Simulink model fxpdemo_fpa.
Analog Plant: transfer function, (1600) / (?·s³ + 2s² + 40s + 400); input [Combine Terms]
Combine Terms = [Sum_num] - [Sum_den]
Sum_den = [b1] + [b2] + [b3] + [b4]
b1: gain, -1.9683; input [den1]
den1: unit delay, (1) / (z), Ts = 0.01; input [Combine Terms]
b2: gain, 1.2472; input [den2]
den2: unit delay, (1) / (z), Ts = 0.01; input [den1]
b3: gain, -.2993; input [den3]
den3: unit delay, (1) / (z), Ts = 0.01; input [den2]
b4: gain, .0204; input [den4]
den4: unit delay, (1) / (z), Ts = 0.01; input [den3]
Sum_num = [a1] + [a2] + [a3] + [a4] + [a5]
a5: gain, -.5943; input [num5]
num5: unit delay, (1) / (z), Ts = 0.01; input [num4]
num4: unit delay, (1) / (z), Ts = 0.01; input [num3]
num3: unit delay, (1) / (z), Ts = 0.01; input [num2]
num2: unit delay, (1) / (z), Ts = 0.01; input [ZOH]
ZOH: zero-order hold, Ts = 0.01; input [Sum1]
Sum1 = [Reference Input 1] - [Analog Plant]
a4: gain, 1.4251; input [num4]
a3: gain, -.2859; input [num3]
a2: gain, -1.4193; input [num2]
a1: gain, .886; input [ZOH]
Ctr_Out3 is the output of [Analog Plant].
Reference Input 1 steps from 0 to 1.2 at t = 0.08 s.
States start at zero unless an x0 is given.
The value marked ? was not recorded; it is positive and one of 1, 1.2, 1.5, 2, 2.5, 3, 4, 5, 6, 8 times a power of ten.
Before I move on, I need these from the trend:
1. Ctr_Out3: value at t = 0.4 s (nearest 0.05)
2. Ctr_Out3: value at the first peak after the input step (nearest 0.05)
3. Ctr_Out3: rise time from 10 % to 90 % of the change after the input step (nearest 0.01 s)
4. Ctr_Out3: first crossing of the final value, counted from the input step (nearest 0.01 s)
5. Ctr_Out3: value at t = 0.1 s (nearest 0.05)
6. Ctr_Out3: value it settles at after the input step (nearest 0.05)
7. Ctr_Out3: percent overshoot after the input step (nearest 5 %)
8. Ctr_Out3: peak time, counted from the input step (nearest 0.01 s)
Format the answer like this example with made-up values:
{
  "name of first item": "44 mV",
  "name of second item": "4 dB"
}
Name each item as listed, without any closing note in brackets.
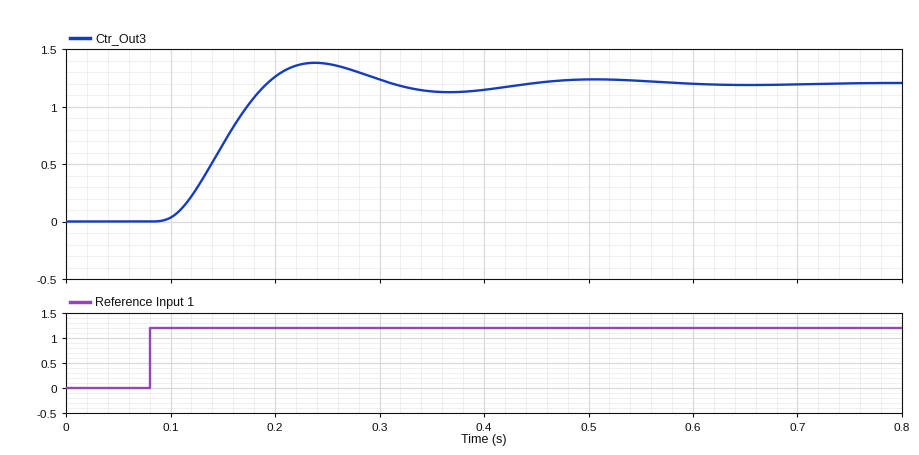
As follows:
{
  "Ctr_Out3: value at t = 0.4 s": "1.15",
  "Ctr_Out3: value at the first peak after the input step": "1.40",
  "Ctr_Out3: rise time from 10 % to 90 % of the change after the input step": "0.07 s",
  "Ctr_Out3: first crossing of the final value, counted from the input step": "0.11 s",
  "Ctr_Out3: value at t = 0.1 s": "0.05",
  "Ctr_Out3: value it settles at after the input step": "1.20",
  "Ctr_Out3: percent overshoot after the input step": "15 %",
  "Ctr_Out3: peak time, counted from the input step": "0.16 s"
}
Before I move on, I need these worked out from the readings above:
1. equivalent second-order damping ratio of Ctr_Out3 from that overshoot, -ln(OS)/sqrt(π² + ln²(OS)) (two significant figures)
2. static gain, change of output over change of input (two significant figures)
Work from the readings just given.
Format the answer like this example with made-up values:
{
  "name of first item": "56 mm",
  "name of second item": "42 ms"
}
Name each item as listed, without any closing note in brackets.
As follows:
{
  "equivalent second-order damping ratio of Ctr_Out3 from that overshoot, -ln(OS)/sqrt(π² + ln²(OS))": "0.52",
  "static gain, change of output over change of input": "1.0"
}
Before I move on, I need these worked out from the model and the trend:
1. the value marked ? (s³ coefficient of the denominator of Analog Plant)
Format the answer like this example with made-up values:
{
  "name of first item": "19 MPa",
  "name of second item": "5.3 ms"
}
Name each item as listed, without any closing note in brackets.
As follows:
{
  "the value marked ?": "0.06"
}
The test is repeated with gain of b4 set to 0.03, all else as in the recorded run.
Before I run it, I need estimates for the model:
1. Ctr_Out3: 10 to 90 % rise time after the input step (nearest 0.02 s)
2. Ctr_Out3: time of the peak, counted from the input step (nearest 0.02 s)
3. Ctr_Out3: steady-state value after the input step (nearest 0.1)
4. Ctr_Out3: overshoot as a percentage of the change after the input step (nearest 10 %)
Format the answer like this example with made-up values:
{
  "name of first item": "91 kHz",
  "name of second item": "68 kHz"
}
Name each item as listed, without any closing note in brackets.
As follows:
{
  "Ctr_Out3: 10 to 90 % rise time after the input step": "0.06 s",
  "Ctr_Out3: time of the peak, counted from the input step": "0.14 s",
  "Ctr_Out3: steady-state value after the input step": "1.0",
  "Ctr_Out3: overshoot as a percentage of the change after the input step": "30 %"
}
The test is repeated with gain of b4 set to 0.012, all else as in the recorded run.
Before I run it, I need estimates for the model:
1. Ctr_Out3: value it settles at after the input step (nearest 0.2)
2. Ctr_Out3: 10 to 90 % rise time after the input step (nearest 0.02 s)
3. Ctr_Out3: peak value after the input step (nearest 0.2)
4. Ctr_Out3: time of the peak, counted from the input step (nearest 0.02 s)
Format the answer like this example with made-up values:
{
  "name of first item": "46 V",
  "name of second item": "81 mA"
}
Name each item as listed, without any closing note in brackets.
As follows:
{
  "Ctr_Out3: value it settles at after the input step": "1.4",
  "Ctr_Out3: 10 to 90 % rise time after the input step": "0.08 s",
  "Ctr_Out3: peak value after the input step": "1.6",
  "Ctr_Out3: time of the peak, counted from the input step": "0.18 s"
}
